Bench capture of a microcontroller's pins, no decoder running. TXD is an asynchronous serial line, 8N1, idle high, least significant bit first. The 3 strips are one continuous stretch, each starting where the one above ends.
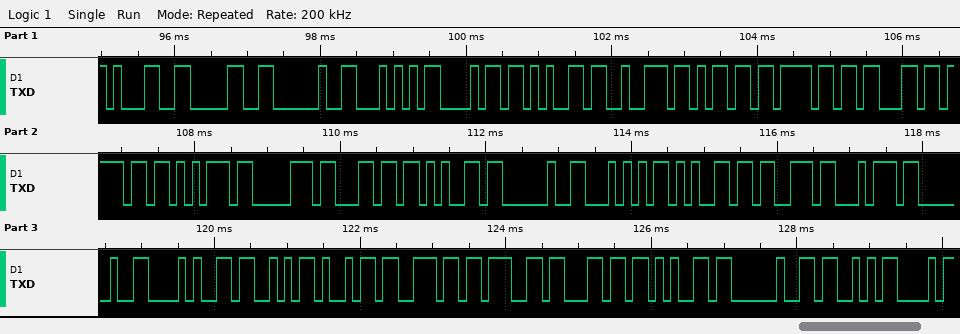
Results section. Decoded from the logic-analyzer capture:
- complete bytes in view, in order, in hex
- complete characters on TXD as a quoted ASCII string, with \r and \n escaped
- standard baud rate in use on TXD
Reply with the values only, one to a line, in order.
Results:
0x31 0x30 0x20 0x54 0x68 0x65 0x72 0x6D 0x6F 0x63 0x6F 0x75 0x70 0x6C 0x65 0x20 0x54 0x65 0x73 0x74 0x20 0x28 0x53 0x69 0x6E 0x67 0x6C 0x65 0x20 0x53
"10 Thermocouple Test (Single S"
9600 baud
